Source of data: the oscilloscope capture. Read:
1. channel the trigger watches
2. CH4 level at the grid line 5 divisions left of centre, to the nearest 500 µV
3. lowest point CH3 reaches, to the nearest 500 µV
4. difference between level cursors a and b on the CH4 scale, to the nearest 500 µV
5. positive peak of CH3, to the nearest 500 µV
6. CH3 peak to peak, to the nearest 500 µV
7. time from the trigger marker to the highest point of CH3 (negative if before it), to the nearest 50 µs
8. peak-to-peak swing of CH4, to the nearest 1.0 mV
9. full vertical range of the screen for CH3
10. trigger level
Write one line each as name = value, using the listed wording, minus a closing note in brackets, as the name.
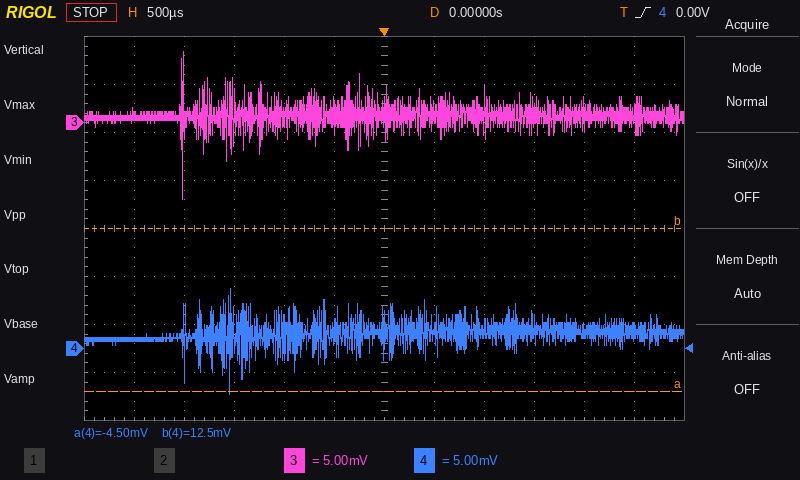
channel the trigger watches = CH4
CH4 level at the grid line 5 divisions left of centre, to the nearest 500 µV = 1.0 mV
lowest point CH3 reaches, to the nearest 500 µV = -8.0 mV
difference between level cursors a and b on the CH4 scale, to the nearest 500 µV = 17.0 mV
positive peak of CH3, to the nearest 500 µV = 7.5 mV
CH3 peak to peak, to the nearest 500 µV = 15.5 mV
time from the trigger marker to the highest point of CH3 (negative if before it), to the nearest 50 µs = -2.00 ms
peak-to-peak swing of CH4, to the nearest 1.0 mV = 11.0 mV
full vertical range of the screen for CH3 = 40 mV
trigger level = 0.00 V
